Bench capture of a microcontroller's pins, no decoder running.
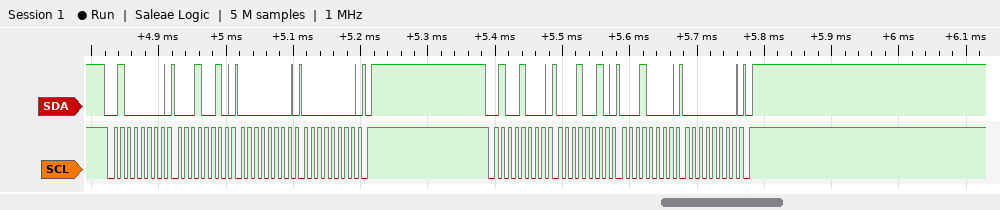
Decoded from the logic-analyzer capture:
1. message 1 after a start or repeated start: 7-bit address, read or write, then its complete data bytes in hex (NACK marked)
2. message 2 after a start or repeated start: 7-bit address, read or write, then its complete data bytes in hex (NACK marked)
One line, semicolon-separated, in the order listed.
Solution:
0x20 write: 12 00 00; 0x24 write: 12 10 00
